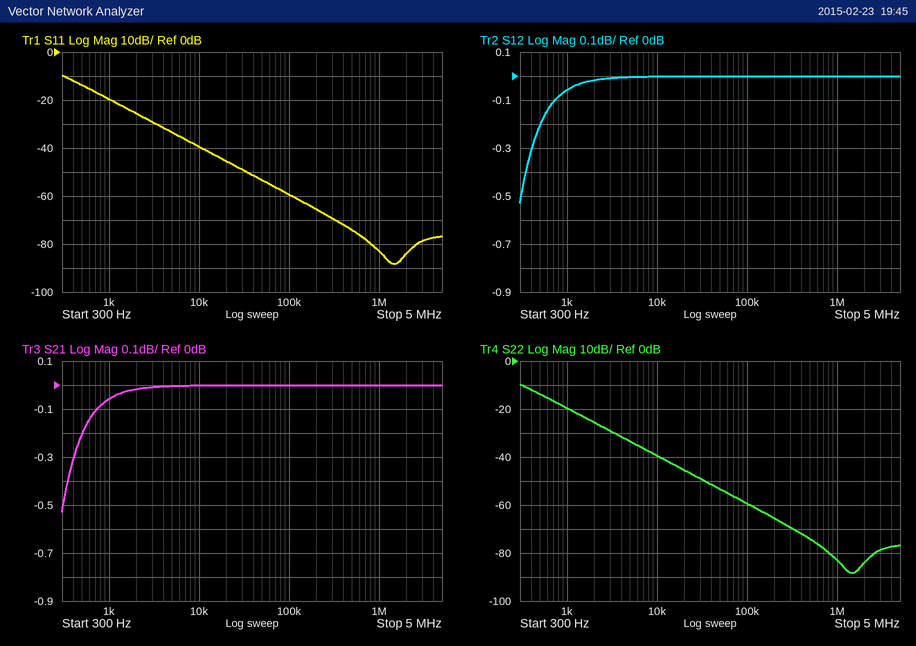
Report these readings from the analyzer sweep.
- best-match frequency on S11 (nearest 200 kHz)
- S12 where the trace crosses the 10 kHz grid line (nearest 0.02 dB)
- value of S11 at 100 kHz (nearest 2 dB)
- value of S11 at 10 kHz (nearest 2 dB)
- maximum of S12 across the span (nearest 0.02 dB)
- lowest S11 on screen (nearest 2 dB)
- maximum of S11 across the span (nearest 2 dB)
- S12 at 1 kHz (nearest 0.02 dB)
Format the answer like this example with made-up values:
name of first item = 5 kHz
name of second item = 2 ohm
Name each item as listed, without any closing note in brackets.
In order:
best-match frequency on S11 = 1.4 MHz
S12 where the trace crosses the 10 kHz grid line = 0.00 dB
value of S11 at 100 kHz = -60 dB
value of S11 at 10 kHz = -40 dB
maximum of S12 across the span = 0.00 dB
lowest S11 on screen = -88 dB
maximum of S11 across the span = -10 dB
S12 at 1 kHz = -0.06 dB
